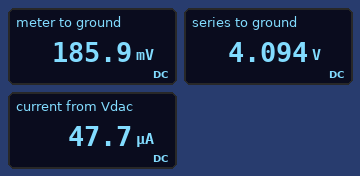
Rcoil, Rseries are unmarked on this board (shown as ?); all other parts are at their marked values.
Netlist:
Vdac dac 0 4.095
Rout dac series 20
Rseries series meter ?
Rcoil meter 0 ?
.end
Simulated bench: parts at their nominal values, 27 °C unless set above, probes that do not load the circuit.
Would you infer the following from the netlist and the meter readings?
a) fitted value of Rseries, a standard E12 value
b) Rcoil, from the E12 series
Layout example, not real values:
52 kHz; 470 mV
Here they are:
82 kΩ; 3.9 kΩ
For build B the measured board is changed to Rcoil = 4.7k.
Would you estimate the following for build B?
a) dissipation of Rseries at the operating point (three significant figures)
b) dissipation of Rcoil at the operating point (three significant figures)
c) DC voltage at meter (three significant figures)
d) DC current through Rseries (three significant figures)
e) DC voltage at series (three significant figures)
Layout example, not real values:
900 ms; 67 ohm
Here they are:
183 µW; 10.5 µW; 222 mV; 47.2 µA; 4.09 V
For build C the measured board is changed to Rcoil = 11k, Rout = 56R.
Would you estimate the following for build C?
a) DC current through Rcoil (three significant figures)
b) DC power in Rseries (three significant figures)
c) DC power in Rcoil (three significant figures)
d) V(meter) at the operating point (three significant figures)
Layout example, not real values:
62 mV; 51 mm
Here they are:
44.0 µA; 159 µW; 21.3 µW; 484 mV
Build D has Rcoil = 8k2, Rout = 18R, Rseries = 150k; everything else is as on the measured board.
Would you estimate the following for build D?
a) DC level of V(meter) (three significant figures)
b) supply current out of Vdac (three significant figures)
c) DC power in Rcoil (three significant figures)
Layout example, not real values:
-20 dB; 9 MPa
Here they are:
212 mV; 25.9 µA; 5.49 µW
